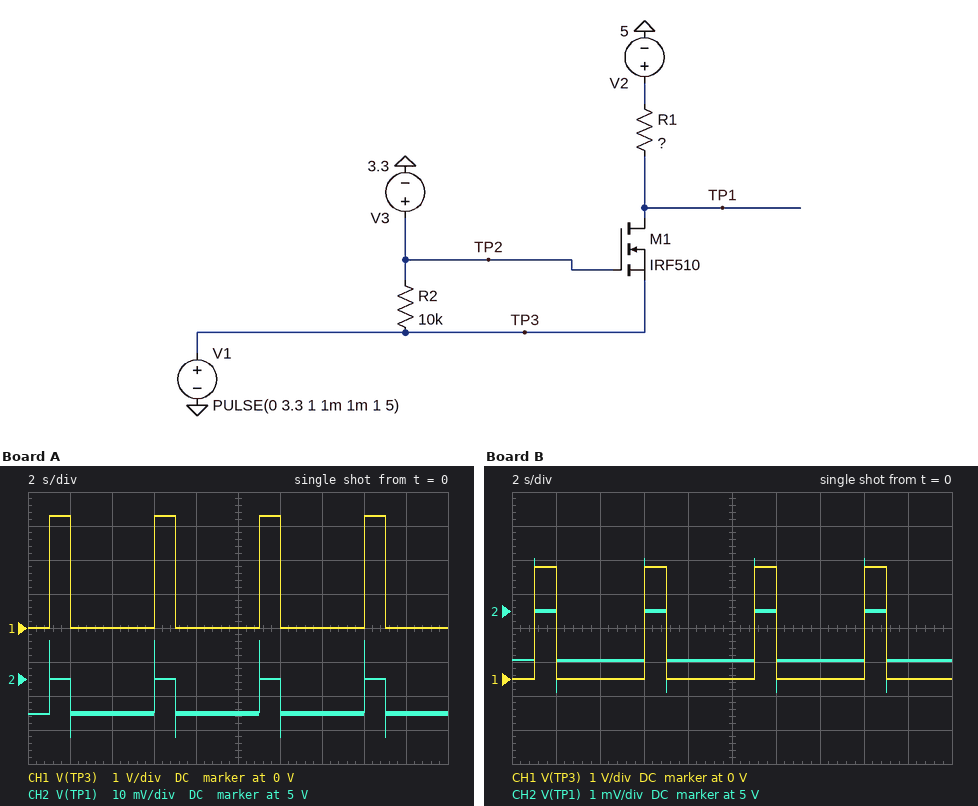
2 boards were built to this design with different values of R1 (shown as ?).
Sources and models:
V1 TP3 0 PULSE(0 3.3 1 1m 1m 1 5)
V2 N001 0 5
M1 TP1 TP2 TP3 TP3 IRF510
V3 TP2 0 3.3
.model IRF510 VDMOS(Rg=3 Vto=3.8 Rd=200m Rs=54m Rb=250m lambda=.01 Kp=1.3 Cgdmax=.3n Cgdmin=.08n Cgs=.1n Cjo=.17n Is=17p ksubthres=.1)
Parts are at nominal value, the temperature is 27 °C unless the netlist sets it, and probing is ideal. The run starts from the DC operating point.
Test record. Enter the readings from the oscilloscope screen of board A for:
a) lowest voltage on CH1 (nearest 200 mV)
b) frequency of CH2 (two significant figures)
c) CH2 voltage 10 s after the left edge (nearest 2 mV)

0 V
200 mHz
4.990 V
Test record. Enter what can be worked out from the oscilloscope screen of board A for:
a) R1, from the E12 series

33 kΩ
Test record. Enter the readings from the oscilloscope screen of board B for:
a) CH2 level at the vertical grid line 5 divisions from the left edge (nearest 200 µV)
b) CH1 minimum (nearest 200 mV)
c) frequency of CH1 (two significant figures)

4.9986 V
0 V
200 mHz
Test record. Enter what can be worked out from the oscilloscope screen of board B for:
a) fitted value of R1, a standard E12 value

4.7 kΩ
